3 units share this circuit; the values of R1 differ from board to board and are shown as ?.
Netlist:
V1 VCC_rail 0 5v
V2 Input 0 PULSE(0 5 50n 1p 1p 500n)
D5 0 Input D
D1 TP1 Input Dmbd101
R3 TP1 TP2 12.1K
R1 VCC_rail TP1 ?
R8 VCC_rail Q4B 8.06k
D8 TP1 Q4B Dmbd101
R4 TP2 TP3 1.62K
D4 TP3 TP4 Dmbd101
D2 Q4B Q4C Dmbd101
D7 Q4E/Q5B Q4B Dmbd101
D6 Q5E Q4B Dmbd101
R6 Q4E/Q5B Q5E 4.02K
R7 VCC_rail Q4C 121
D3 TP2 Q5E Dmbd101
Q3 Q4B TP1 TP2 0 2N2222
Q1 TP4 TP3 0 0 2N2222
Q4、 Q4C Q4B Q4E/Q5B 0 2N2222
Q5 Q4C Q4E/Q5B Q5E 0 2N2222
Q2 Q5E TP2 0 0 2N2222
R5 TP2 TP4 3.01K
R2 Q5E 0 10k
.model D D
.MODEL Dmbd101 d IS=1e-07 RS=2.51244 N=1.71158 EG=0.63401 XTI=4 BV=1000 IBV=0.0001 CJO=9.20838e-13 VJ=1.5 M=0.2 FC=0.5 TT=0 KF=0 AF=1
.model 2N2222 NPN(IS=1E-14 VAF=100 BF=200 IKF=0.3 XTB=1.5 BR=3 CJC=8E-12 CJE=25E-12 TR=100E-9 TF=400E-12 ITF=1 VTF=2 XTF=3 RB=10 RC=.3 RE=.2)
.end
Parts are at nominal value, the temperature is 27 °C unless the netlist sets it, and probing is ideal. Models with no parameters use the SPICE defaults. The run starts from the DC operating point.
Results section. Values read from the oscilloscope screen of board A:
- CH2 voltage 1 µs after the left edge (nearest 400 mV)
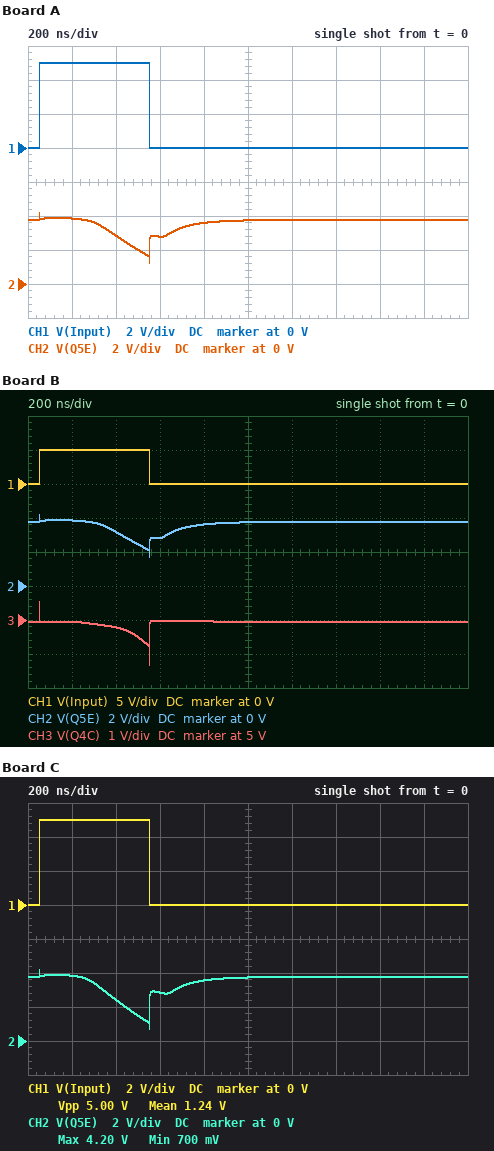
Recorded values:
3.6 V
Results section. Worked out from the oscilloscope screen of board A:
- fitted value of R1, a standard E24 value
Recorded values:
36 kΩ
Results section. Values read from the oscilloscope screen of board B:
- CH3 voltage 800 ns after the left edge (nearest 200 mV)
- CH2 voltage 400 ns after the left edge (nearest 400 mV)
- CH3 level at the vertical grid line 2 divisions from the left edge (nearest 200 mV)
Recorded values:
5.0 V
3.2 V
4.8 V
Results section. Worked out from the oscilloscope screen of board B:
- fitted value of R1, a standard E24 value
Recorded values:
39 kΩ
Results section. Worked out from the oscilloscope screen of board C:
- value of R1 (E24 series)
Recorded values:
33 kΩ
